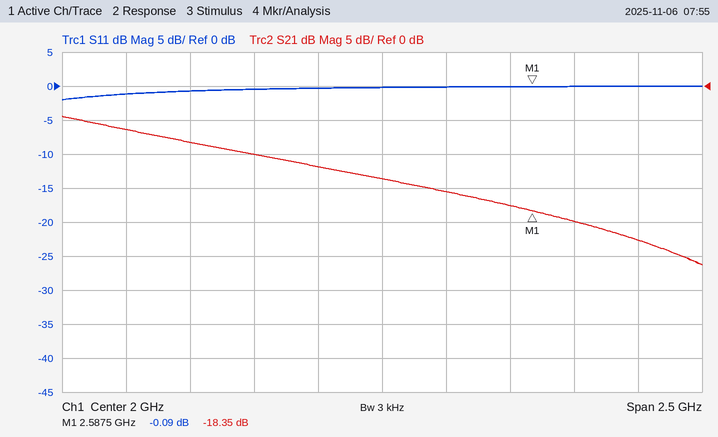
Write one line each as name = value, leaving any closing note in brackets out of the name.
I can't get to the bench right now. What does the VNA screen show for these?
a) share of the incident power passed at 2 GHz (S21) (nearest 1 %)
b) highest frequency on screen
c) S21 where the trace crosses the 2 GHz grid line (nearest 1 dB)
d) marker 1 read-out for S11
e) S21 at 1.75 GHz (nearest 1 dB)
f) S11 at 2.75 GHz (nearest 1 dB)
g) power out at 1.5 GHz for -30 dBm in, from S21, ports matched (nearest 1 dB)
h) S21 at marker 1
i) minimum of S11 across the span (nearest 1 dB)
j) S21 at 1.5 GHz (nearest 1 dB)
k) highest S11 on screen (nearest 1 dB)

share of the incident power passed at 2 GHz (S21) = 4 %
highest frequency on screen = 3.25 GHz
S21 where the trace crosses the 2 GHz grid line = -14 dB
marker 1 read-out for S11 = -0.09 dB
S21 at 1.75 GHz = -12 dB
S11 at 2.75 GHz = 0 dB
power out at 1.5 GHz for -30 dBm in, from S21, ports matched = -40 dBm
S21 at marker 1 = -18.35 dB
minimum of S11 across the span = -2 dB
S21 at 1.5 GHz = -10 dB
highest S11 on screen = 0 dB
